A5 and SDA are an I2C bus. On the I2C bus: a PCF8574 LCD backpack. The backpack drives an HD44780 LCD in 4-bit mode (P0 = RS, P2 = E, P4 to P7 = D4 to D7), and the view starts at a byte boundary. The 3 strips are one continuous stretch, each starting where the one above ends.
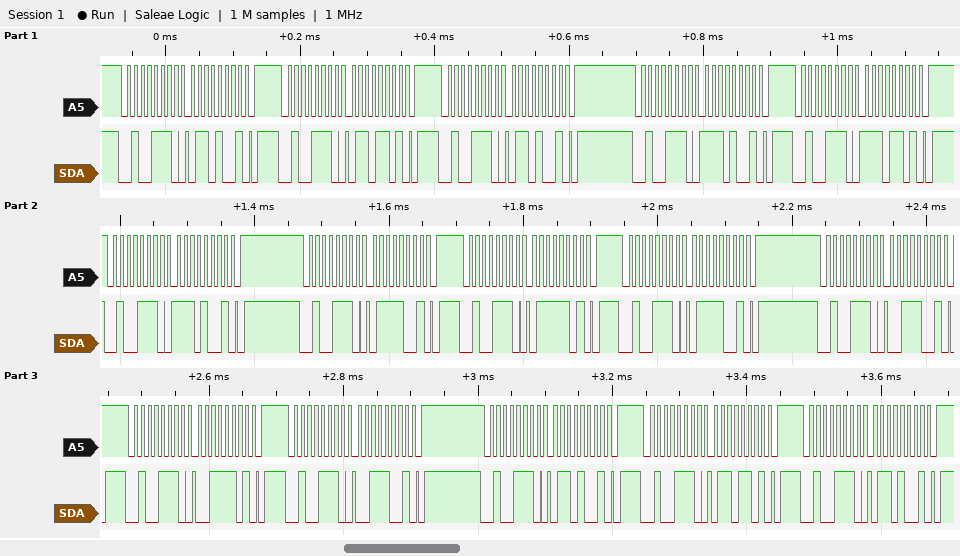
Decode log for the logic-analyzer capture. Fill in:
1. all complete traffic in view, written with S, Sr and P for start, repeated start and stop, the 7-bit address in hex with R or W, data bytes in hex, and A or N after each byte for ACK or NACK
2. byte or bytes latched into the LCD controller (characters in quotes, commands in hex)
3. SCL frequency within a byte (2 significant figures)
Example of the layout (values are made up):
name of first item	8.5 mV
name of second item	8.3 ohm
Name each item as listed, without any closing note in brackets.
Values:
all complete traffic in view, written with S, Sr and P for start, repeated start and stop, the 7-bit address in hex with R or W, data bytes in hex, and A or N after each byte for ACK or NACK	S 27W A 69 A P S 27W A 6D A P S 27W A 69 A P S 27W A E9 A P S 27W A ED A P S 27W A E9 A P S 27W A 79 A P S 27W A 7D A P S 27W A 79 A P S 27W A 39 A P S 27W A 3D A P S 27W A 39 A P S 27W A 69 A P S 27W A 6D A P S 27W A 69 A P
byte or bytes latched into the LCD controller	'n' 's'
SCL frequency within a byte	100 kHz
